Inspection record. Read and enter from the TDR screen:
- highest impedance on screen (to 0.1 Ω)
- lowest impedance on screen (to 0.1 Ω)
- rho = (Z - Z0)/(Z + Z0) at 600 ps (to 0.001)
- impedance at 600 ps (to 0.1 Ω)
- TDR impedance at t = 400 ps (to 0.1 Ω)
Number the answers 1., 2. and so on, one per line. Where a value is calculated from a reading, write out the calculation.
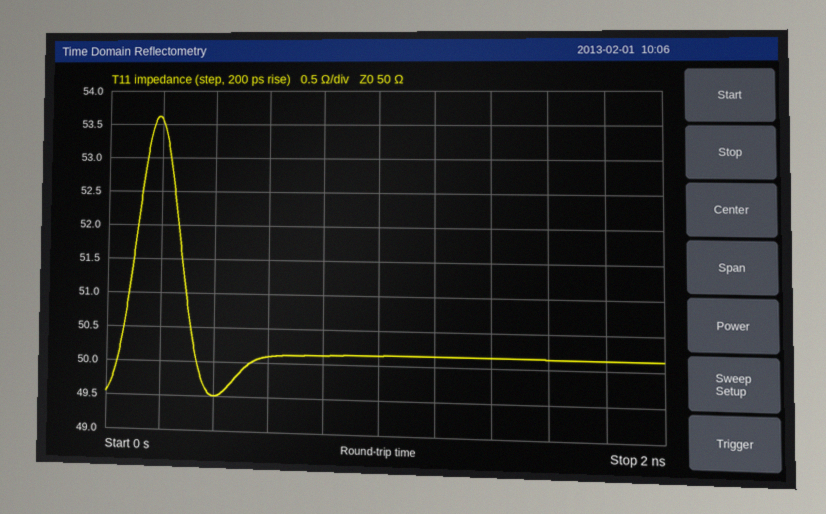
1. 53.6 Ω
2. 49.5 Ω
3. (50.1 − 50)/(50.1 + 50) ≈ +0.001
4. 50.1 Ω
5. 49.5 Ω
